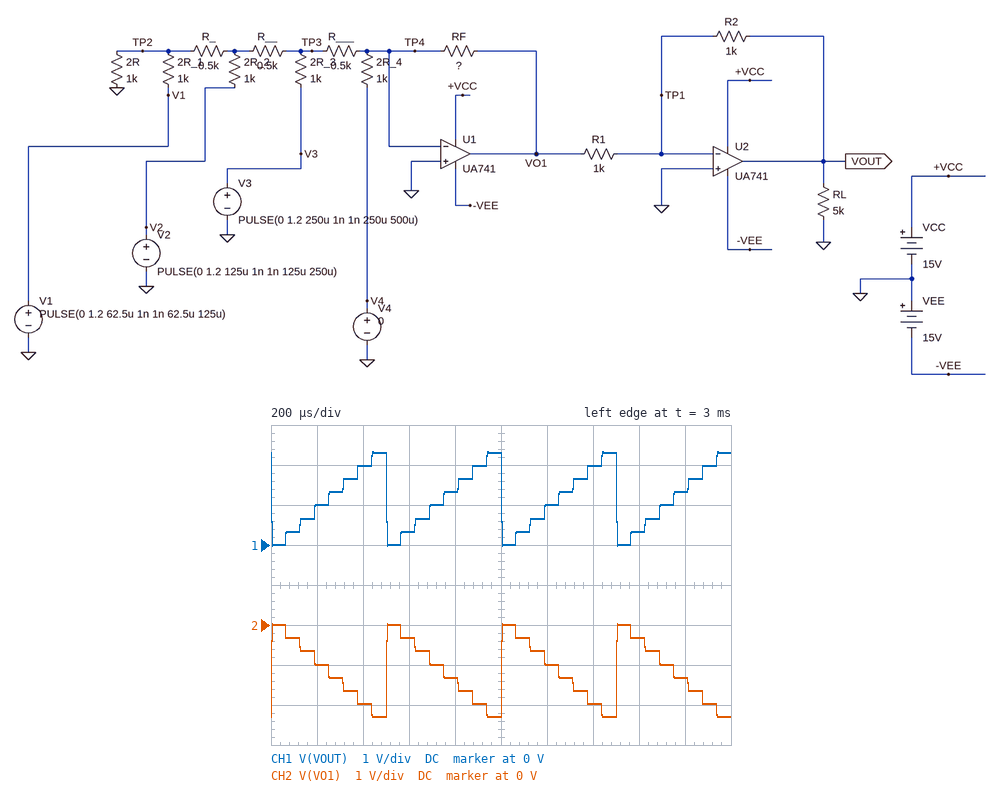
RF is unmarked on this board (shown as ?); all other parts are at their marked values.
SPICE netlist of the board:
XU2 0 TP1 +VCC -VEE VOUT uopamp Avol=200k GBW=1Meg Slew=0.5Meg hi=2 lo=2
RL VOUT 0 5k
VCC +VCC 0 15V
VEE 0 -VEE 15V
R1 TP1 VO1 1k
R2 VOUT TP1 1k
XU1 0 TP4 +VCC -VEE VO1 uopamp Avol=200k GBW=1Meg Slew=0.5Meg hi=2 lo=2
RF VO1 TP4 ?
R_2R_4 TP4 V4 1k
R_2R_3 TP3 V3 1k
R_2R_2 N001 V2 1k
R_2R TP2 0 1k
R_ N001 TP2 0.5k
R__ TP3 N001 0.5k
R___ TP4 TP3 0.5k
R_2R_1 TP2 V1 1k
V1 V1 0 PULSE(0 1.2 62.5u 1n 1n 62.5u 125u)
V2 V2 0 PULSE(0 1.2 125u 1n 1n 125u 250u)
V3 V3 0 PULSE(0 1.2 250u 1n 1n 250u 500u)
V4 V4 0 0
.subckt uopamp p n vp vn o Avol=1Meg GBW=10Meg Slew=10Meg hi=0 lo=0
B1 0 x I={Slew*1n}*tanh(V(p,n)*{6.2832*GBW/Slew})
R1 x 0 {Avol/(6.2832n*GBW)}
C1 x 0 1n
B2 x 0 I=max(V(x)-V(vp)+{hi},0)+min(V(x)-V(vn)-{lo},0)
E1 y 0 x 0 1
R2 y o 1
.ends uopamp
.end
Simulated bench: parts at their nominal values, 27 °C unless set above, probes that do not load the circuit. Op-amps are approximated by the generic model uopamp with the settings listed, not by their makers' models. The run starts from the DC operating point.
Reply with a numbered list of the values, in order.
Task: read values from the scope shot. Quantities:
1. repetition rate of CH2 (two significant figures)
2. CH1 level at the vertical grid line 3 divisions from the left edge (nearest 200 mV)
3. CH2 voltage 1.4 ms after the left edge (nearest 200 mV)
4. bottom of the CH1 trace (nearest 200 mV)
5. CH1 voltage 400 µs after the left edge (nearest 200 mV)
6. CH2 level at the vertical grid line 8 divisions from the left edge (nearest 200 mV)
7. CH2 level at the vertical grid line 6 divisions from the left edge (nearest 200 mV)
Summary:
1. 2.0 kHz
2. 400 mV
3. -2.0 V
4. 0 V
5. 2.0 V
6. -400 mV
7. -1.0 V
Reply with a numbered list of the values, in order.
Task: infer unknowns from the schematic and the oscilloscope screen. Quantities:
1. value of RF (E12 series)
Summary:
1. 2.2 kΩ
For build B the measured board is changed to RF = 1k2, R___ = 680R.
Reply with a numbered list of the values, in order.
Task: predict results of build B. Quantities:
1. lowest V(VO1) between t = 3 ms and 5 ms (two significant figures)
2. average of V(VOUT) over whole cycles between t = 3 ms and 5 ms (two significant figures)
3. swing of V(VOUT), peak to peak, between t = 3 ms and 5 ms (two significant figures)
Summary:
1. -1.1 V
2. 540 mV
3. 1.1 V
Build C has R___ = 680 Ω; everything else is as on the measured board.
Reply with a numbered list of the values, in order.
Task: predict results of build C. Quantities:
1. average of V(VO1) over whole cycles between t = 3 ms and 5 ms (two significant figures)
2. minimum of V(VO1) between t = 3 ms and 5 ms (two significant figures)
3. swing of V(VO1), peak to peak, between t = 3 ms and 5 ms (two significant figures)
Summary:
1. -980 mV
2. -2.0 V
3. 2.0 V
